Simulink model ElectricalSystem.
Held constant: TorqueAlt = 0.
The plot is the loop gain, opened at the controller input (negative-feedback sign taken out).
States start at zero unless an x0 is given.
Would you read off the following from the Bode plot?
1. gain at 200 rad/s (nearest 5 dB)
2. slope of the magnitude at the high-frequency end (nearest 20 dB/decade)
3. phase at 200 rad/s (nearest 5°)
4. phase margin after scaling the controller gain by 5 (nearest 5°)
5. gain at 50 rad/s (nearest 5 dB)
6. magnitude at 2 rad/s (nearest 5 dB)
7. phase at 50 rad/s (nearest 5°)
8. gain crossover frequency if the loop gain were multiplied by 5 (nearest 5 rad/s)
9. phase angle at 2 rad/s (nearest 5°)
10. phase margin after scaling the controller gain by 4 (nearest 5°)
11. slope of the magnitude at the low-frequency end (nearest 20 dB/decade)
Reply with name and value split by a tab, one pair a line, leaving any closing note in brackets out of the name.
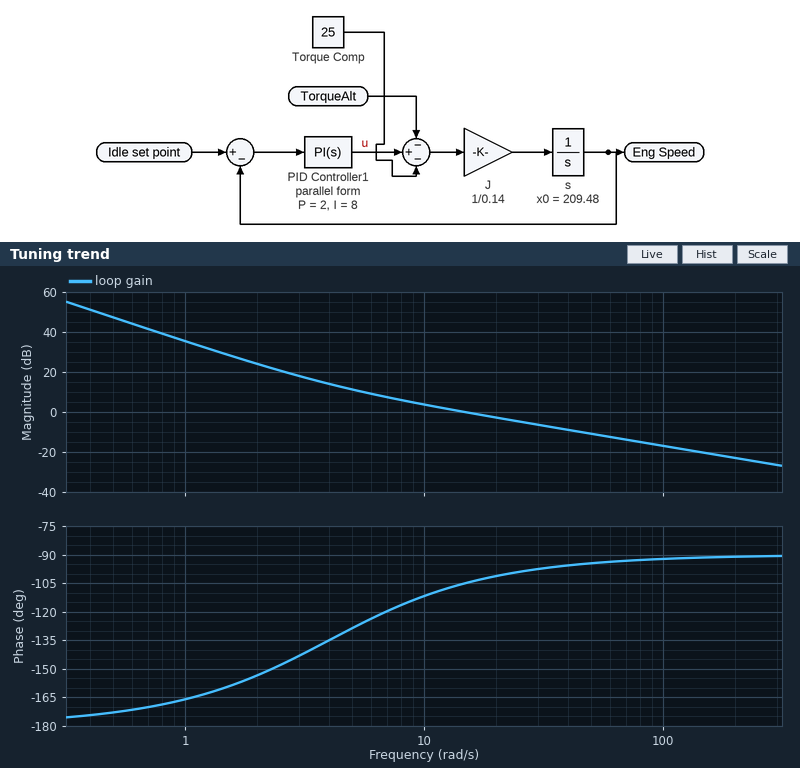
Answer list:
gain at 200 rad/s	-25 dB
slope of the magnitude at the high-frequency end	-20 dB/decade
phase at 200 rad/s	-90°
phase margin after scaling the controller gain by 5	85°
gain at 50 rad/s	-10 dB
magnitude at 2 rad/s	25 dB
phase at 50 rad/s	-95°
gain crossover frequency if the loop gain were multiplied by 5	70 rad/s
phase angle at 2 rad/s	-155°
phase margin after scaling the controller gain by 4	85°
slope of the magnitude at the low-frequency end	-40 dB/decade
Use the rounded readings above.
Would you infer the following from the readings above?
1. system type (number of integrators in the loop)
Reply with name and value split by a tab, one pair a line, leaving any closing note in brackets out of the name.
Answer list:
system type	2
